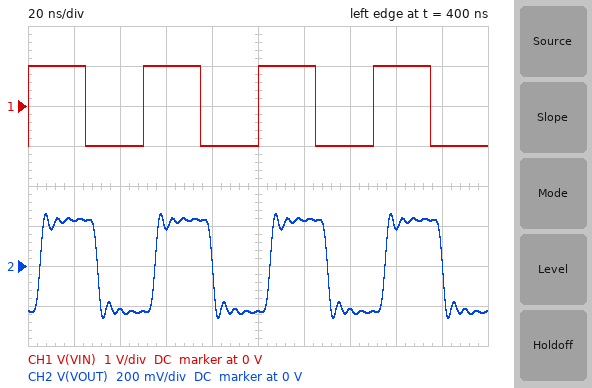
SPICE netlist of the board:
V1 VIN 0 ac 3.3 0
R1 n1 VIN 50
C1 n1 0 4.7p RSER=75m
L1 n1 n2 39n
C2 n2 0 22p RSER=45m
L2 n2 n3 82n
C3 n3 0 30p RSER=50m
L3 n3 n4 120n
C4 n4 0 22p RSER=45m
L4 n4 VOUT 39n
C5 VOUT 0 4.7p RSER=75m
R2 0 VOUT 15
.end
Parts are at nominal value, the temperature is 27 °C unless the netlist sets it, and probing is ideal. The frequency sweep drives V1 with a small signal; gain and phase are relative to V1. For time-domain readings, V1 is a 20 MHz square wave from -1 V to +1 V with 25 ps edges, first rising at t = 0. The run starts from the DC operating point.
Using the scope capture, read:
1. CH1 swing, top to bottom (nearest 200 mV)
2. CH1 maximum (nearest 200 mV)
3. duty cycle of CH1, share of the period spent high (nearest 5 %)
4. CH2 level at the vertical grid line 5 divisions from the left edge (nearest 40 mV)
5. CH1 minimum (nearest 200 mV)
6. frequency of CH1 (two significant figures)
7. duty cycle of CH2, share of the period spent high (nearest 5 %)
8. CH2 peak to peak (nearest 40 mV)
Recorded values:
2.0 V
1.0 V
50 %
-240 mV
-1.0 V
20 MHz
50 %
520 mV
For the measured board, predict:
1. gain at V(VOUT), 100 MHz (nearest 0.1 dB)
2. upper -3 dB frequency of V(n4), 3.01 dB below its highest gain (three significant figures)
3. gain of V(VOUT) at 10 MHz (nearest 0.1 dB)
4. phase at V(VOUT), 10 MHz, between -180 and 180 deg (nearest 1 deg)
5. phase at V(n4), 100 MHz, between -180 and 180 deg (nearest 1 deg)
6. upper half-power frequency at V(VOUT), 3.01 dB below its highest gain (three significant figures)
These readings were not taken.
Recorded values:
-14.0 dB
213 MHz
-12.8 dB
-19 deg
-117 deg
198 MHz
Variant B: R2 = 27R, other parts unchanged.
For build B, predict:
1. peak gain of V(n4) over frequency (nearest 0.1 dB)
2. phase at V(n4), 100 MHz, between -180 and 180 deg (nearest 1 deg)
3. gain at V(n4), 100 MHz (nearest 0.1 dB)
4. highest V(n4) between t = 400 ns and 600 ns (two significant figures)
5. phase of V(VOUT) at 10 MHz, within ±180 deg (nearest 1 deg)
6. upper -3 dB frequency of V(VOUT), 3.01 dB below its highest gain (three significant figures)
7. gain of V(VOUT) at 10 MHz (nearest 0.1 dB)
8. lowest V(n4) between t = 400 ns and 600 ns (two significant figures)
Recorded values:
-6.8 dB
-134 deg
-7.7 dB
540 mV
-18 deg
175 MHz
-9.1 dB
-540 mV
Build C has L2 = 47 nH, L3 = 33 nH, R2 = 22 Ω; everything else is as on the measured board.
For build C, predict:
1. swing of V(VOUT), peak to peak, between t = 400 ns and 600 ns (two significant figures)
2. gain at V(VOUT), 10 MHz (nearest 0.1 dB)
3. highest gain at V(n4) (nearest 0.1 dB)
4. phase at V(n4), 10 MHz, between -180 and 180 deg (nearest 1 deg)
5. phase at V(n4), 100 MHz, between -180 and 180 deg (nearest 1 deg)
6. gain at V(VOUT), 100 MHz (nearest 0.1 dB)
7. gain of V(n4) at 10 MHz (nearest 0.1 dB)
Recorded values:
850 mV
-10.3 dB
-0.5 dB
-6 deg
-86 deg
-9.8 dB
-10.2 dB
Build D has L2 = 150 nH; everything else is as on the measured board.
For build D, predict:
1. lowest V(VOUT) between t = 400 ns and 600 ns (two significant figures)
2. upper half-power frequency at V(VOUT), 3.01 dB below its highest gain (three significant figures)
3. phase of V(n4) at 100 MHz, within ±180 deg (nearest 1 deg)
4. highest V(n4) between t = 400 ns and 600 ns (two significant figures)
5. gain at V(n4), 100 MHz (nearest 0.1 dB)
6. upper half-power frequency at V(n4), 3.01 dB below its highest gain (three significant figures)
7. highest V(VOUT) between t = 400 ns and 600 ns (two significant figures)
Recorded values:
-250 mV
123 MHz
-142 deg
430 mV
-6.5 dB
131 MHz
250 mV
